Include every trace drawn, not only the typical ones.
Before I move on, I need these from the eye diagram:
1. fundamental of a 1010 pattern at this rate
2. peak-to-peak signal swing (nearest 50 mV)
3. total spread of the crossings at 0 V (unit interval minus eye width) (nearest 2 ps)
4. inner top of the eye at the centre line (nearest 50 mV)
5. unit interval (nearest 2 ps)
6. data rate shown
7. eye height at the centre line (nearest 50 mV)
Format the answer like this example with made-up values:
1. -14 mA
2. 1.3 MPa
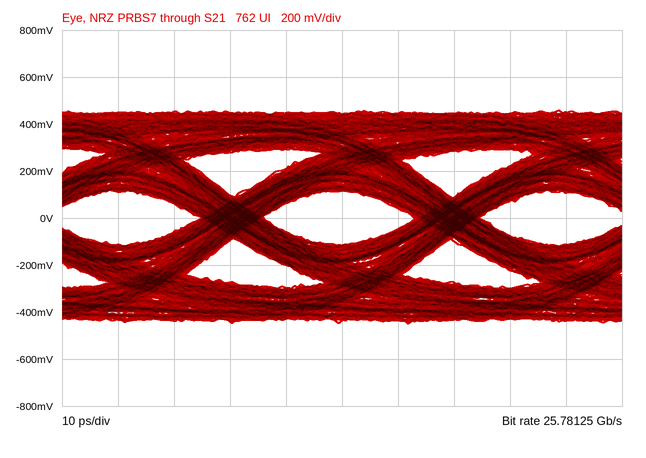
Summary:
1. 12.89062 GHz
2. 900 mV
3. 12 ps
4. 100 mV
5. 38 ps
6. 25.78125 Gb/s
7. 250 mV
